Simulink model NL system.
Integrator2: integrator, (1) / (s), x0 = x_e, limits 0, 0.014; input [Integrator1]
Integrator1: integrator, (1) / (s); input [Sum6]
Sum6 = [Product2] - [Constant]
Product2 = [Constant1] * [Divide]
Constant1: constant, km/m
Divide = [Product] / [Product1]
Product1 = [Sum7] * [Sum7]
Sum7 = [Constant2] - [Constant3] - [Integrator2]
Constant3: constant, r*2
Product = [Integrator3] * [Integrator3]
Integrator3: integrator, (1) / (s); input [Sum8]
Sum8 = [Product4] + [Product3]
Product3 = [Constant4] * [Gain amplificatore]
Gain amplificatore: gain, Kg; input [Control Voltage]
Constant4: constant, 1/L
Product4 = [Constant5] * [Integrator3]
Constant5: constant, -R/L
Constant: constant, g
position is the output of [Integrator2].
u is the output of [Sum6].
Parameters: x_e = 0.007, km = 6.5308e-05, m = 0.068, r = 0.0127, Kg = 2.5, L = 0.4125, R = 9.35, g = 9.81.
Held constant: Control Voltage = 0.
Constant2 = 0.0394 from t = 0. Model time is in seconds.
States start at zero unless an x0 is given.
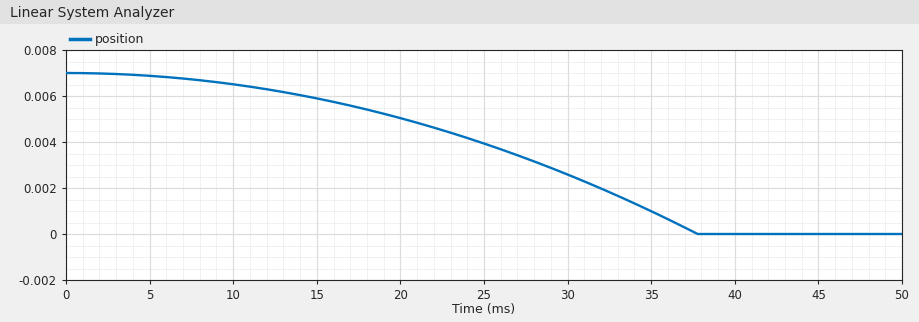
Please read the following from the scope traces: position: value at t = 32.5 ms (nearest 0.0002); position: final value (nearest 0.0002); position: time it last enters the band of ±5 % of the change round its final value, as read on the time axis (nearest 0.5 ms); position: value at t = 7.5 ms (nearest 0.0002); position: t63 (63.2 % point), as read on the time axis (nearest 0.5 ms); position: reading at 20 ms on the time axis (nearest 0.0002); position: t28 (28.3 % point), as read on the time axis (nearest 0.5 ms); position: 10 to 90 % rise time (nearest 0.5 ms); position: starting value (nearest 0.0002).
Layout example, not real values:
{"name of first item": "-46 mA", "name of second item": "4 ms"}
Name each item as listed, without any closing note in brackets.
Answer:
{"position: value at t = 32.5 ms": "0.0018", "position: final value": "0.0000", "position: time it last enters the band of ±5 % of the change round its final value, as read on the time axis": "37.0 ms", "position: value at t = 7.5 ms": "0.0068", "position: t63 (63.2 % point), as read on the time axis": "30.0 ms", "position: reading at 20 ms on the time axis": "0.0050", "position: t28 (28.3 % point), as read on the time axis": "20.0 ms", "position: 10 to 90 % rise time": "24.0 ms", "position: starting value": "0.0070"}
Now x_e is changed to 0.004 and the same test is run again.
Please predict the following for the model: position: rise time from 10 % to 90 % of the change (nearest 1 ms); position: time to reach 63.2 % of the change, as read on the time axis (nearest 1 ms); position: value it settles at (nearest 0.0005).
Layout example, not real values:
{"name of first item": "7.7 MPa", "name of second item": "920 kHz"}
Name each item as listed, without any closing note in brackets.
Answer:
{"position: rise time from 10 % to 90 % of the change": "18 ms", "position: time to reach 63.2 % of the change, as read on the time axis": "23 ms", "position: value it settles at": "0.0000"}
